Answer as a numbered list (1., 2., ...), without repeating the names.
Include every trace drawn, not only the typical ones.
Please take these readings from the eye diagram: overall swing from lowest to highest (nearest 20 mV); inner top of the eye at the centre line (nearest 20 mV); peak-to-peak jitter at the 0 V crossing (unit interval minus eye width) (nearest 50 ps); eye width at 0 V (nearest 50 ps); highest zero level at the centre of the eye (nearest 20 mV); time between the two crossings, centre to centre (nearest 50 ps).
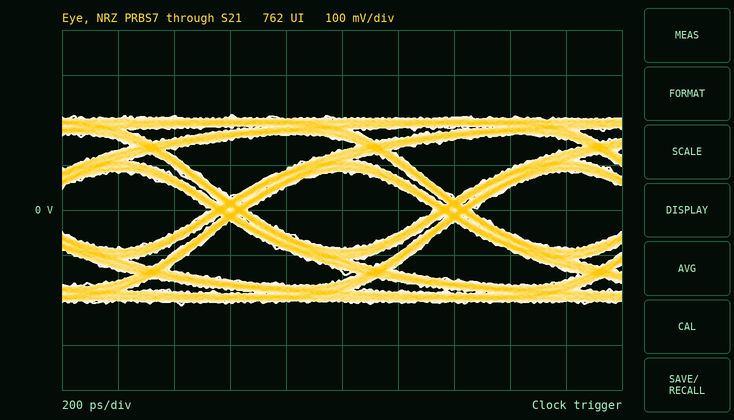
1. 420 mV
2. 80 mV
3. 150 ps
4. 650 ps
5. -80 mV
6. 800 ps
